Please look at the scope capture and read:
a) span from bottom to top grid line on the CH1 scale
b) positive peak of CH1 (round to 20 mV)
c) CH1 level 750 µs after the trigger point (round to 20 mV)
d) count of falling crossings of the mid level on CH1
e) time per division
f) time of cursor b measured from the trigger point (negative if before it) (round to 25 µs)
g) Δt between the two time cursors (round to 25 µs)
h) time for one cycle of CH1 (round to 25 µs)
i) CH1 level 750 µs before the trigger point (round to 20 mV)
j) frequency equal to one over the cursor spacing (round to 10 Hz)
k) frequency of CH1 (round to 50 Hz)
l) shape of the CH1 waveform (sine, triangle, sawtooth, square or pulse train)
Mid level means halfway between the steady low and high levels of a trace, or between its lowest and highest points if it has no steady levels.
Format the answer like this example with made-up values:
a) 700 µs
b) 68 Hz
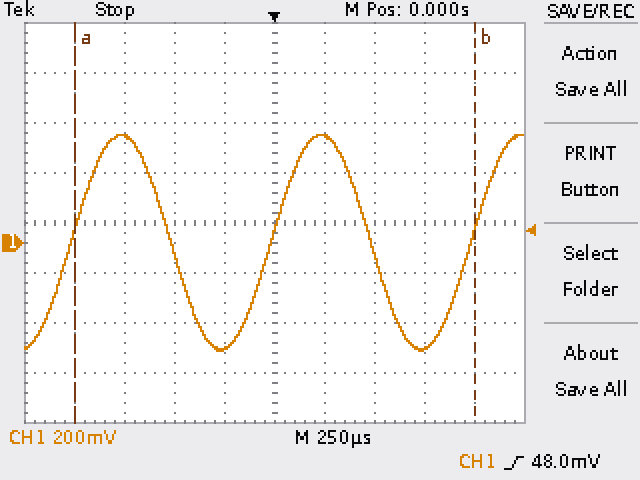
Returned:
a) 1.6 V
b) 440 mV
c) -420 mV
d) 2
e) 250 µs
f) +1.000 ms
g) 2.000 ms
h) 1.000 ms
i) 420 mV
j) 500 Hz
k) 1.00 kHz
l) sine
